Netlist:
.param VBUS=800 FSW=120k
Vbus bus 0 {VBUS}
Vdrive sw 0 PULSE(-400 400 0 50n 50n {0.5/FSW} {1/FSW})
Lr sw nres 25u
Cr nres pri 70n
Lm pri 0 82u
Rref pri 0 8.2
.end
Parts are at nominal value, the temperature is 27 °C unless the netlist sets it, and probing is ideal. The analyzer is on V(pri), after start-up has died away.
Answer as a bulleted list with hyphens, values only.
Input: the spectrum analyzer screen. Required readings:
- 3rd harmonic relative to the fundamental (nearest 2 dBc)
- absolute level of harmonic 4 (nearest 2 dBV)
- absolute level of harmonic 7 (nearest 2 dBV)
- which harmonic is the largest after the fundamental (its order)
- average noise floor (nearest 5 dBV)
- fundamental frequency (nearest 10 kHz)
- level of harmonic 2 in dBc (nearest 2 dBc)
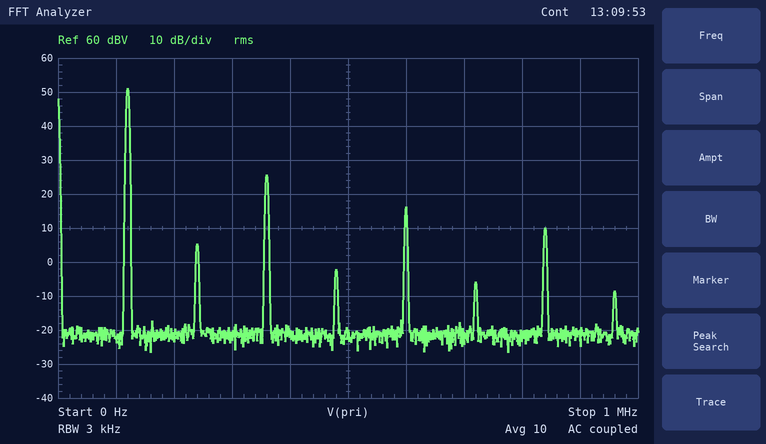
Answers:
- -26 dBc
- -2 dBV
- 10 dBV
- 3
- -20 dBV
- 120 kHz
- -46 dBc
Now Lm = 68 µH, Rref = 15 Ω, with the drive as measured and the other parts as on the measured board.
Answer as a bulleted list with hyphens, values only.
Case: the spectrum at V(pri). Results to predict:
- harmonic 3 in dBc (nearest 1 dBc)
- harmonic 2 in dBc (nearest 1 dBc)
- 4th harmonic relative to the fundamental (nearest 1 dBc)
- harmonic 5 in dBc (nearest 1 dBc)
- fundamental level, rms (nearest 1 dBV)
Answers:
- -21 dBc
- -42 dBc
- -48 dBc
- -30 dBc
- 51 dBV
